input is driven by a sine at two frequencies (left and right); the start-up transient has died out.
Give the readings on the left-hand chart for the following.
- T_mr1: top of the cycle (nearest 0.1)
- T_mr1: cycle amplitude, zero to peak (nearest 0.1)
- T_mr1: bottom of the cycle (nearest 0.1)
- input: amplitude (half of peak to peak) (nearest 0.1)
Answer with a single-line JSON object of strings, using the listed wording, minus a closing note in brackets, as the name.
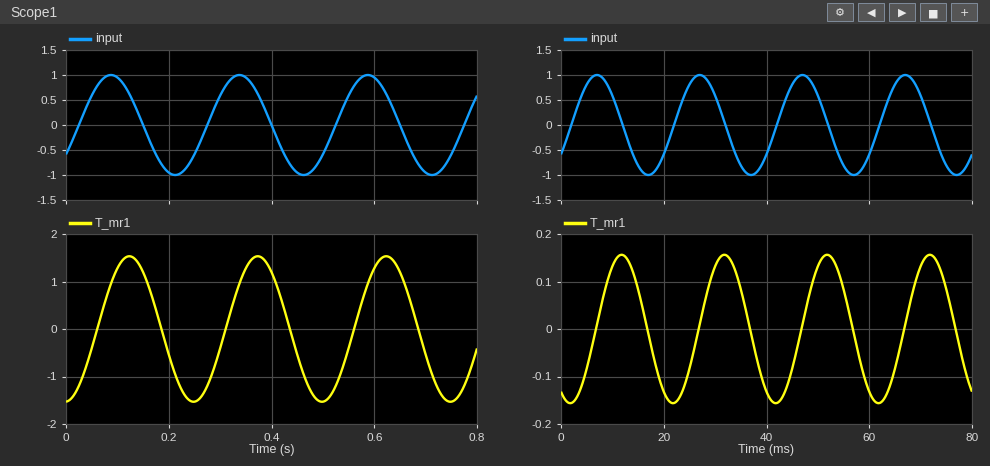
{"T_mr1: top of the cycle": "1.5", "T_mr1: cycle amplitude, zero to peak": "1.5", "T_mr1: bottom of the cycle": "-1.5", "input: amplitude (half of peak to peak)": "1.0"}
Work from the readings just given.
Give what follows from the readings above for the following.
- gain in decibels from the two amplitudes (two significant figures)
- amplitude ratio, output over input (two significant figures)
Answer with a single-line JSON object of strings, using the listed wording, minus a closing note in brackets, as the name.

{"gain in decibels from the two amplitudes": "3.5 dB", "amplitude ratio, output over input": "1.5"}
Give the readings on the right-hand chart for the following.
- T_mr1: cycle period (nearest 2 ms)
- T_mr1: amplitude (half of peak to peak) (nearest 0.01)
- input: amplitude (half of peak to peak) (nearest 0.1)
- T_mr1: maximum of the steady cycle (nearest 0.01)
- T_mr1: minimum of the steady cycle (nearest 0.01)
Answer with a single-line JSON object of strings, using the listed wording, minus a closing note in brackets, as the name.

{"T_mr1: cycle period": "20 ms", "T_mr1: amplitude (half of peak to peak)": "0.16", "input: amplitude (half of peak to peak)": "1.0", "T_mr1: maximum of the steady cycle": "0.16", "T_mr1: minimum of the steady cycle": "-0.16"}
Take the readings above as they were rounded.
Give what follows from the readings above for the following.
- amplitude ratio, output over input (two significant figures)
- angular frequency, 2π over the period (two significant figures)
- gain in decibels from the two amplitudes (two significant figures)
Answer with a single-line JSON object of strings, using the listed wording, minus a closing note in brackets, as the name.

{"amplitude ratio, output over input": "0.16", "angular frequency, 2π over the period": "0.31 rad/ms", "gain in decibels from the two amplitudes": "-16 dB"}
